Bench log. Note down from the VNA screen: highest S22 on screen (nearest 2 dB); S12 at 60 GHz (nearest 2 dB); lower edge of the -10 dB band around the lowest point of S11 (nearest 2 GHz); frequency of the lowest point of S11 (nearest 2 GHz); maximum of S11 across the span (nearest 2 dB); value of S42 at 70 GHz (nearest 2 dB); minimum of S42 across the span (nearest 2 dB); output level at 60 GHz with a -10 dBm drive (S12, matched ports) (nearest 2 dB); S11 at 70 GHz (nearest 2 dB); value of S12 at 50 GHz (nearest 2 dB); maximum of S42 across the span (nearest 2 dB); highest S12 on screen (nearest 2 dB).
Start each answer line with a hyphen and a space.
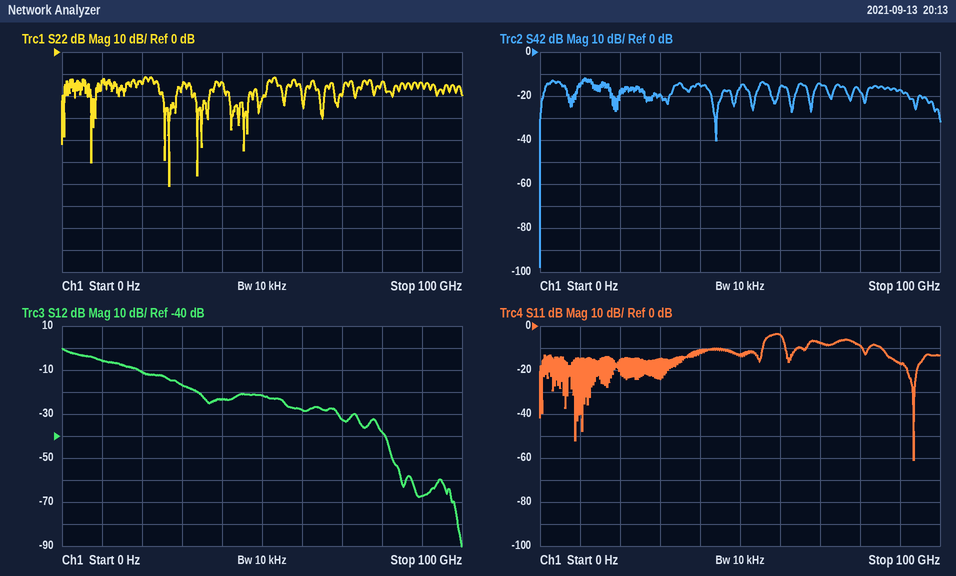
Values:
- -12 dB
- -28 dB
- 86 GHz
- 94 GHz
- -4 dB
- -14 dB
- -98 dB
- -38 dBm
- -8 dB
- -22 dB
- -12 dB
- 0 dB
